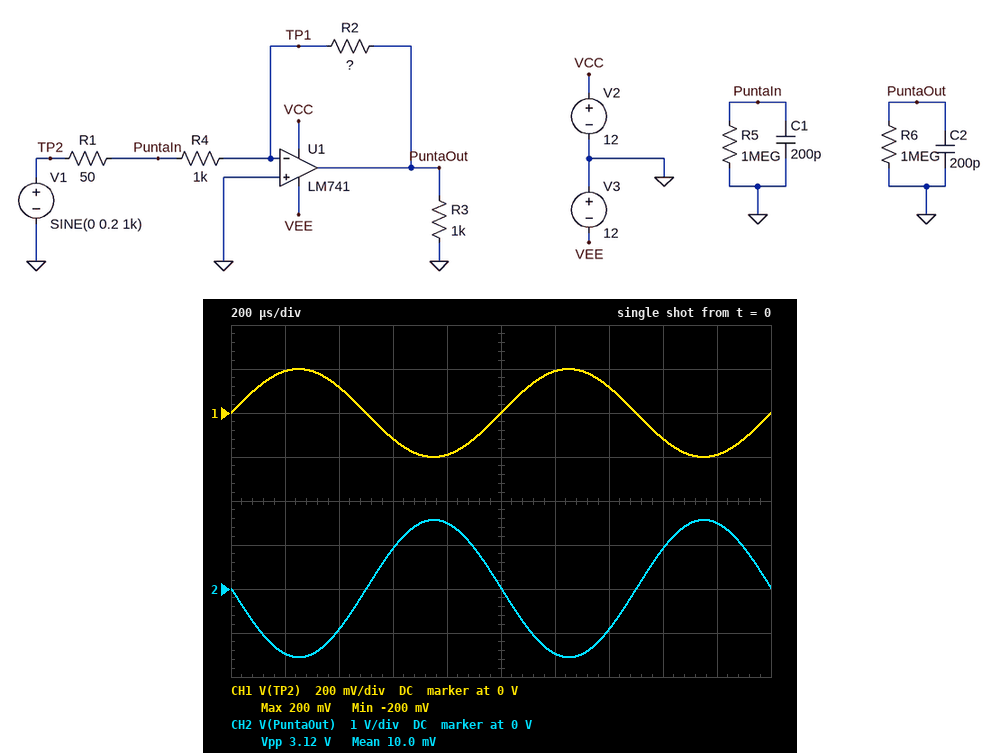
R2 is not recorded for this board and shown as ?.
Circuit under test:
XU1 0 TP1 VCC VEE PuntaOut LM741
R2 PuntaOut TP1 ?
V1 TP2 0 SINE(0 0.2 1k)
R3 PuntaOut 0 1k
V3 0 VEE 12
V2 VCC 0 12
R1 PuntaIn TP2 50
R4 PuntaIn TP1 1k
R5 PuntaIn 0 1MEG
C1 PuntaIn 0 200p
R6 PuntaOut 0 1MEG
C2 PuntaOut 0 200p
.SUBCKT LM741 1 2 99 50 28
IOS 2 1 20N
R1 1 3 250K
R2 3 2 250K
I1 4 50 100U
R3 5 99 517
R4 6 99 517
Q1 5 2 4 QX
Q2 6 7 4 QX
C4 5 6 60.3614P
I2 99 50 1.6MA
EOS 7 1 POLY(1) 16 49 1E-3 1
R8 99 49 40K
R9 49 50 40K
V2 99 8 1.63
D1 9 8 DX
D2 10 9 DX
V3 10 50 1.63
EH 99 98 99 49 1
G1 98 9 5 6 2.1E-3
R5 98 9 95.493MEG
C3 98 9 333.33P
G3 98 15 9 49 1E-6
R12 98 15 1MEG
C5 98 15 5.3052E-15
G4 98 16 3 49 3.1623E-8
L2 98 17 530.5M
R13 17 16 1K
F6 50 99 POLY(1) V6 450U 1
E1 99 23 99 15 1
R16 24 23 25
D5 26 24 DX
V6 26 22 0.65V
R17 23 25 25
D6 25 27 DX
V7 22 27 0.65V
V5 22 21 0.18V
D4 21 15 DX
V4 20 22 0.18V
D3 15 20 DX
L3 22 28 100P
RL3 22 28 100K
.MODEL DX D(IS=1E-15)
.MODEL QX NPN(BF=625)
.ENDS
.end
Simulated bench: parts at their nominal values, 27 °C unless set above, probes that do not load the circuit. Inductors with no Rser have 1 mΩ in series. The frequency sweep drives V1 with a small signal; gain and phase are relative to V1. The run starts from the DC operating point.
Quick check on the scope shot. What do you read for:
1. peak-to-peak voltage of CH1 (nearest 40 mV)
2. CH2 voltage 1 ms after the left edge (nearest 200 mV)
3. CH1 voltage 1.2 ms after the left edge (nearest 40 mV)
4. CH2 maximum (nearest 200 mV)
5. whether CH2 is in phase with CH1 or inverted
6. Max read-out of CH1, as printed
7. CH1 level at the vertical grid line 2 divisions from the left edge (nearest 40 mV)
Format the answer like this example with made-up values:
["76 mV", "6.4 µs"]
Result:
["400 mV", "0 V", "200 mV", "1.6 V", "inverted", "200 mV", "120 mV"]
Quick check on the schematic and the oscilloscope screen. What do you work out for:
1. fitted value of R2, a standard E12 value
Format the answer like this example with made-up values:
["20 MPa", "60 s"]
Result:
["8.2 kΩ"]
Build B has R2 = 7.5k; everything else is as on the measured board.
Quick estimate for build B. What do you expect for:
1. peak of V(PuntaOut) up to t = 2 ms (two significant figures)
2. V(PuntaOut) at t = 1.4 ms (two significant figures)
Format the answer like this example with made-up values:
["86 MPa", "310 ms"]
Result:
["1.4 V", "-840 mV"]
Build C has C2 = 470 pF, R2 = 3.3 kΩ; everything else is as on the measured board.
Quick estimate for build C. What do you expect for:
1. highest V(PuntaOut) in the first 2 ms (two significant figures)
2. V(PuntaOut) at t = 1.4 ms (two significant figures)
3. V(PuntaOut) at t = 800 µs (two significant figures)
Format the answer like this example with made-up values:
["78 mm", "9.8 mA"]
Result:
["630 mV", "-370 mV", "600 mV"]
